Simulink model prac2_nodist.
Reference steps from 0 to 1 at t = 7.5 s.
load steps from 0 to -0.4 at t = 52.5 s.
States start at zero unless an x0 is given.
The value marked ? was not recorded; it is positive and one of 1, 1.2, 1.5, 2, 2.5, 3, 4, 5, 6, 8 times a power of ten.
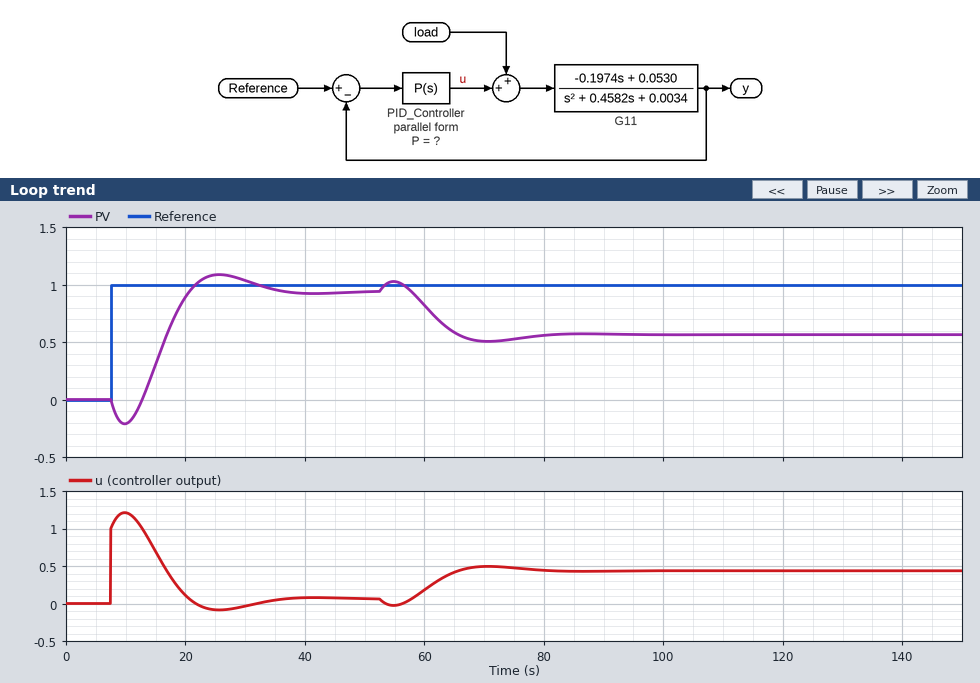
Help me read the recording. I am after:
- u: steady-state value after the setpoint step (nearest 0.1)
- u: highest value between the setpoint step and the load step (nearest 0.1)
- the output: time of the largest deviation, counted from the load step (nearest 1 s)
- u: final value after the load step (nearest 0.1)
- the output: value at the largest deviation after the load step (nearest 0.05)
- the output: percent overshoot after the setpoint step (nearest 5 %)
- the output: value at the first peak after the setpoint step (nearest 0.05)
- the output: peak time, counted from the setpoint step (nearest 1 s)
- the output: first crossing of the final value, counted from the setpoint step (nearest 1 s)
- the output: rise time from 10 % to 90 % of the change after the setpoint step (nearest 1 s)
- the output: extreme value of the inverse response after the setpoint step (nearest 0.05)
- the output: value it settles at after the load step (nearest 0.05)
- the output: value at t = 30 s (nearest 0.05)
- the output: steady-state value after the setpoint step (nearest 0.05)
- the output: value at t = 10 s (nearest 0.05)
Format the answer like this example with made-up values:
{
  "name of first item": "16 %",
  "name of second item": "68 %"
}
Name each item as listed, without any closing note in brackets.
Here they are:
{
  "u: steady-state value after the setpoint step": "0.1",
  "u: highest value between the setpoint step and the load step": "1.2",
  "the output: time of the largest deviation, counted from the load step": "18 s",
  "u: final value after the load step": "0.4",
  "the output: value at the largest deviation after the load step": "0.50",
  "the output: percent overshoot after the setpoint step": "15 %",
  "the output: value at the first peak after the setpoint step": "1.10",
  "the output: peak time, counted from the setpoint step": "18 s",
  "the output: first crossing of the final value, counted from the setpoint step": "13 s",
  "the output: rise time from 10 % to 90 % of the change after the setpoint step": "6 s",
  "the output: extreme value of the inverse response after the setpoint step": "-0.20",
  "the output: value it settles at after the load step": "0.55",
  "the output: value at t = 30 s": "1.05",
  "the output: steady-state value after the setpoint step": "0.95",
  "the output: value at t = 10 s": "-0.20"
}
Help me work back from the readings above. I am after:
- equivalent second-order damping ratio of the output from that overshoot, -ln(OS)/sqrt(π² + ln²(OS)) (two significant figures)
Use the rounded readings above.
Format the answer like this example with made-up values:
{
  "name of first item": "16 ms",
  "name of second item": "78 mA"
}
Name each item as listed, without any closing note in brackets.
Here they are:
{
  "equivalent second-order damping ratio of the output from that overshoot, -ln(OS)/sqrt(π² + ln²(OS))": "0.52"
}
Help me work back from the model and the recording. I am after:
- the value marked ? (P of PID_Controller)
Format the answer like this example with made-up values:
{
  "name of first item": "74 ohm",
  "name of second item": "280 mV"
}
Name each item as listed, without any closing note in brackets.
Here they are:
{
  "the value marked ?": "1"
}
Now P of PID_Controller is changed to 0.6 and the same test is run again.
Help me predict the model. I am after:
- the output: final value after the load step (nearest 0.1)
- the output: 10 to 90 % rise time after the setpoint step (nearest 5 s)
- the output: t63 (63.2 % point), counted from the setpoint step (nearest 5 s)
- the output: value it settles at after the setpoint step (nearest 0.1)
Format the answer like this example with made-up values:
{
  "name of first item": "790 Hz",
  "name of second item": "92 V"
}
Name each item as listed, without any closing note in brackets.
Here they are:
{
  "the output: final value after the load step": "0.3",
  "the output: 10 to 90 % rise time after the setpoint step": "15 s",
  "the output: t63 (63.2 % point), counted from the setpoint step": "15 s",
  "the output: value it settles at after the setpoint step": "0.9"
}
